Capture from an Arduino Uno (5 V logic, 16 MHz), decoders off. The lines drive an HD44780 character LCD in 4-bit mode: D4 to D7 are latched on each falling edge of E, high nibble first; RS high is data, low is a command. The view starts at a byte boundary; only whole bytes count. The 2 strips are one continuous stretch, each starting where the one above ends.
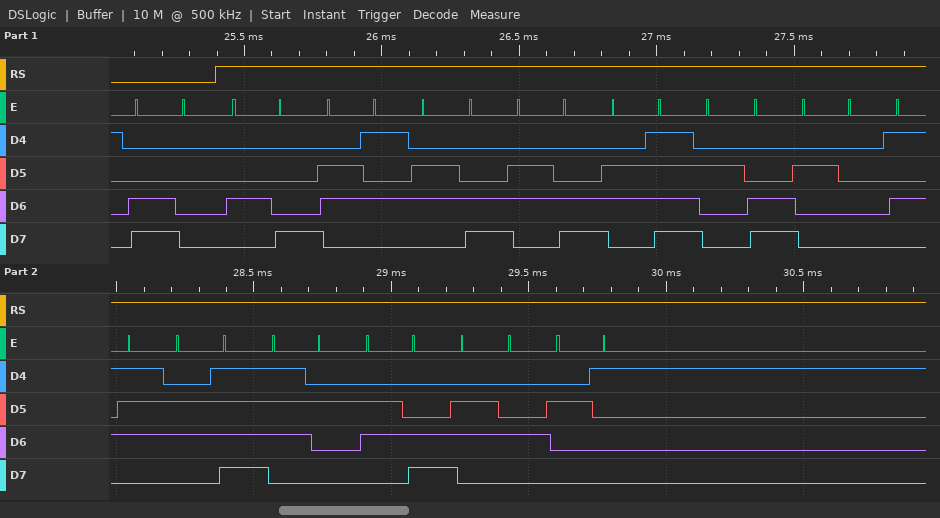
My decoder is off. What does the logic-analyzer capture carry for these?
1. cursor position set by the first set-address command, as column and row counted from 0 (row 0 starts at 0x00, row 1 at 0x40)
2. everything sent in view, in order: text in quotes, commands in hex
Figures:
column 0, row 1
0xC0 "Hello, World!"
